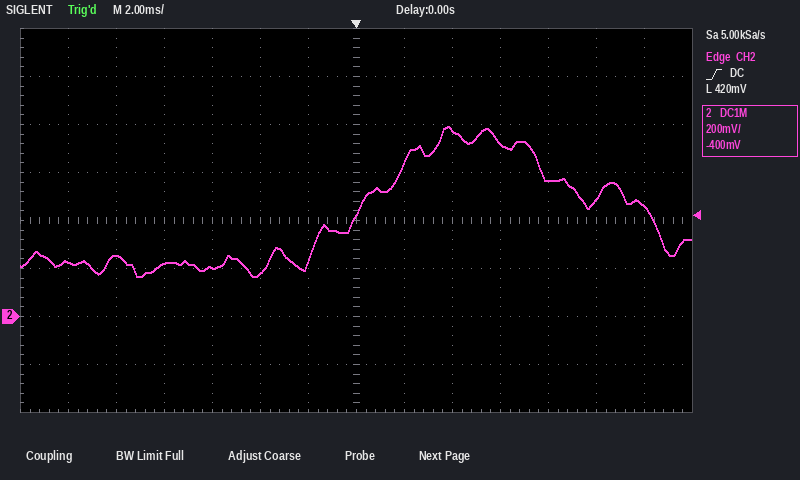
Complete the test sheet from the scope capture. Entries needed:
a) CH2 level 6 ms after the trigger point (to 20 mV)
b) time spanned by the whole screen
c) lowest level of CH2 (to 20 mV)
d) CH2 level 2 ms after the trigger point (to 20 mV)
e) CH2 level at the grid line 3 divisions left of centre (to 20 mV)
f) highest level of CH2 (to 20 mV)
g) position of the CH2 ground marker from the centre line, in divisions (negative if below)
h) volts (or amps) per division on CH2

720 mV
28 ms
160 mV
640 mV
200 mV
800 mV
-2.0 div
200 mV
